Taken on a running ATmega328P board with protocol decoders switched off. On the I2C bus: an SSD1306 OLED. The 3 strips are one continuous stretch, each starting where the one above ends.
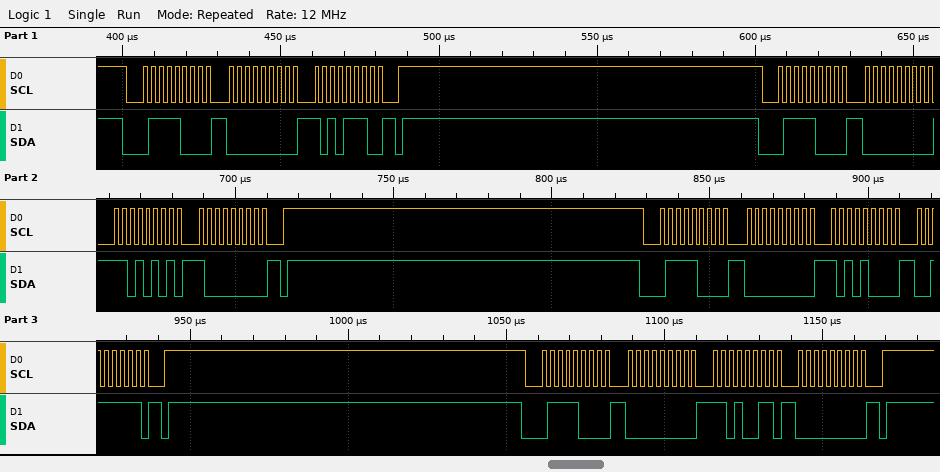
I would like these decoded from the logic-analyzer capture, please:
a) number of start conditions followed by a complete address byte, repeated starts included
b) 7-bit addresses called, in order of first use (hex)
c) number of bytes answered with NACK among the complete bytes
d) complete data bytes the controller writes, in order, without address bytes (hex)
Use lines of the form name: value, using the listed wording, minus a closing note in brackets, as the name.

number of start conditions followed by a complete address byte, repeated starts included: 4
7-bit addresses called, in order of first use: 0x3C
number of bytes answered with NACK among the complete bytes: 0
complete data bytes the controller writes, in order, without address bytes: 00 AE 00 D5 80 00 A8 3F 00 D3 00
